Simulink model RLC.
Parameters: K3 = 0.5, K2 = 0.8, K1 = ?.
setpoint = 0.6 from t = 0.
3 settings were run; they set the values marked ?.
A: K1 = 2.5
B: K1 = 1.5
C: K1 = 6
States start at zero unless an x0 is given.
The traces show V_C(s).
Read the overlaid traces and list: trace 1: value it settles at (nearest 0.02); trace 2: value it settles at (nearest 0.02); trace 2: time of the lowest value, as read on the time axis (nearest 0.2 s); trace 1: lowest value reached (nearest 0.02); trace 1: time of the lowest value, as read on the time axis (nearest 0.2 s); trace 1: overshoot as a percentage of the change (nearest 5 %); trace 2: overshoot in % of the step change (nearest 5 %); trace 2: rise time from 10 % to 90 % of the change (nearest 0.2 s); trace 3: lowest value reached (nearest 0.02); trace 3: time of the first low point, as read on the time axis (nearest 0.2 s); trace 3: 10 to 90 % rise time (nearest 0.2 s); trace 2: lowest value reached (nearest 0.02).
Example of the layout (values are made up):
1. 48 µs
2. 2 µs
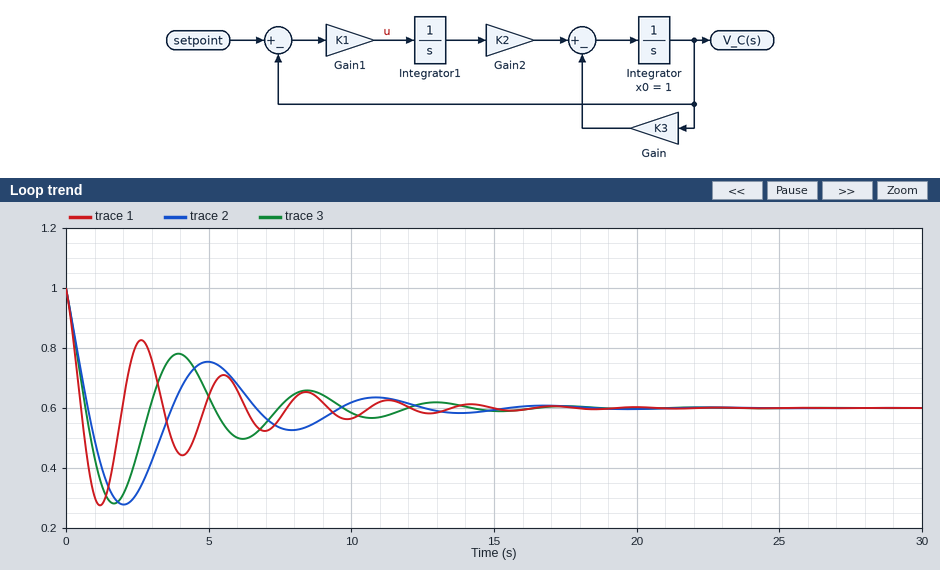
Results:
1. 0.60
2. 0.60
3. 2.0 s
4. 0.28
5. 1.2 s
6. 80 %
7. 80 %
8. 0.6 s
9. 0.28
10. 1.6 s
11. 0.6 s
12. 0.28
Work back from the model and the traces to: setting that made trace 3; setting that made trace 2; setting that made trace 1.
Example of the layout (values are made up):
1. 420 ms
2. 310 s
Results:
1. A
2. B
3. C
